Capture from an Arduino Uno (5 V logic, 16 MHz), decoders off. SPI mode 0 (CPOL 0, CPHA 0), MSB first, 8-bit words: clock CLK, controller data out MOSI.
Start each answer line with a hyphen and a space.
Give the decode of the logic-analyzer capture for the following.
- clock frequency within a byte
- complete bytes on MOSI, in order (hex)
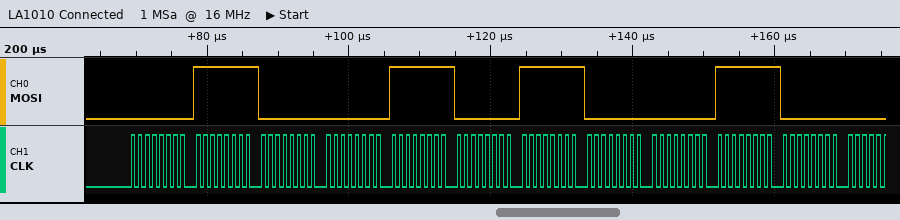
- 1 MHz
- 0x00 0xFF 0x00 0x00 0xFF 0x00 0xFF 0x00 0x00 0xFF 0x00
